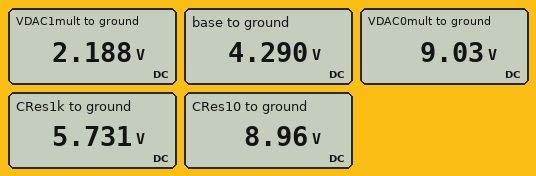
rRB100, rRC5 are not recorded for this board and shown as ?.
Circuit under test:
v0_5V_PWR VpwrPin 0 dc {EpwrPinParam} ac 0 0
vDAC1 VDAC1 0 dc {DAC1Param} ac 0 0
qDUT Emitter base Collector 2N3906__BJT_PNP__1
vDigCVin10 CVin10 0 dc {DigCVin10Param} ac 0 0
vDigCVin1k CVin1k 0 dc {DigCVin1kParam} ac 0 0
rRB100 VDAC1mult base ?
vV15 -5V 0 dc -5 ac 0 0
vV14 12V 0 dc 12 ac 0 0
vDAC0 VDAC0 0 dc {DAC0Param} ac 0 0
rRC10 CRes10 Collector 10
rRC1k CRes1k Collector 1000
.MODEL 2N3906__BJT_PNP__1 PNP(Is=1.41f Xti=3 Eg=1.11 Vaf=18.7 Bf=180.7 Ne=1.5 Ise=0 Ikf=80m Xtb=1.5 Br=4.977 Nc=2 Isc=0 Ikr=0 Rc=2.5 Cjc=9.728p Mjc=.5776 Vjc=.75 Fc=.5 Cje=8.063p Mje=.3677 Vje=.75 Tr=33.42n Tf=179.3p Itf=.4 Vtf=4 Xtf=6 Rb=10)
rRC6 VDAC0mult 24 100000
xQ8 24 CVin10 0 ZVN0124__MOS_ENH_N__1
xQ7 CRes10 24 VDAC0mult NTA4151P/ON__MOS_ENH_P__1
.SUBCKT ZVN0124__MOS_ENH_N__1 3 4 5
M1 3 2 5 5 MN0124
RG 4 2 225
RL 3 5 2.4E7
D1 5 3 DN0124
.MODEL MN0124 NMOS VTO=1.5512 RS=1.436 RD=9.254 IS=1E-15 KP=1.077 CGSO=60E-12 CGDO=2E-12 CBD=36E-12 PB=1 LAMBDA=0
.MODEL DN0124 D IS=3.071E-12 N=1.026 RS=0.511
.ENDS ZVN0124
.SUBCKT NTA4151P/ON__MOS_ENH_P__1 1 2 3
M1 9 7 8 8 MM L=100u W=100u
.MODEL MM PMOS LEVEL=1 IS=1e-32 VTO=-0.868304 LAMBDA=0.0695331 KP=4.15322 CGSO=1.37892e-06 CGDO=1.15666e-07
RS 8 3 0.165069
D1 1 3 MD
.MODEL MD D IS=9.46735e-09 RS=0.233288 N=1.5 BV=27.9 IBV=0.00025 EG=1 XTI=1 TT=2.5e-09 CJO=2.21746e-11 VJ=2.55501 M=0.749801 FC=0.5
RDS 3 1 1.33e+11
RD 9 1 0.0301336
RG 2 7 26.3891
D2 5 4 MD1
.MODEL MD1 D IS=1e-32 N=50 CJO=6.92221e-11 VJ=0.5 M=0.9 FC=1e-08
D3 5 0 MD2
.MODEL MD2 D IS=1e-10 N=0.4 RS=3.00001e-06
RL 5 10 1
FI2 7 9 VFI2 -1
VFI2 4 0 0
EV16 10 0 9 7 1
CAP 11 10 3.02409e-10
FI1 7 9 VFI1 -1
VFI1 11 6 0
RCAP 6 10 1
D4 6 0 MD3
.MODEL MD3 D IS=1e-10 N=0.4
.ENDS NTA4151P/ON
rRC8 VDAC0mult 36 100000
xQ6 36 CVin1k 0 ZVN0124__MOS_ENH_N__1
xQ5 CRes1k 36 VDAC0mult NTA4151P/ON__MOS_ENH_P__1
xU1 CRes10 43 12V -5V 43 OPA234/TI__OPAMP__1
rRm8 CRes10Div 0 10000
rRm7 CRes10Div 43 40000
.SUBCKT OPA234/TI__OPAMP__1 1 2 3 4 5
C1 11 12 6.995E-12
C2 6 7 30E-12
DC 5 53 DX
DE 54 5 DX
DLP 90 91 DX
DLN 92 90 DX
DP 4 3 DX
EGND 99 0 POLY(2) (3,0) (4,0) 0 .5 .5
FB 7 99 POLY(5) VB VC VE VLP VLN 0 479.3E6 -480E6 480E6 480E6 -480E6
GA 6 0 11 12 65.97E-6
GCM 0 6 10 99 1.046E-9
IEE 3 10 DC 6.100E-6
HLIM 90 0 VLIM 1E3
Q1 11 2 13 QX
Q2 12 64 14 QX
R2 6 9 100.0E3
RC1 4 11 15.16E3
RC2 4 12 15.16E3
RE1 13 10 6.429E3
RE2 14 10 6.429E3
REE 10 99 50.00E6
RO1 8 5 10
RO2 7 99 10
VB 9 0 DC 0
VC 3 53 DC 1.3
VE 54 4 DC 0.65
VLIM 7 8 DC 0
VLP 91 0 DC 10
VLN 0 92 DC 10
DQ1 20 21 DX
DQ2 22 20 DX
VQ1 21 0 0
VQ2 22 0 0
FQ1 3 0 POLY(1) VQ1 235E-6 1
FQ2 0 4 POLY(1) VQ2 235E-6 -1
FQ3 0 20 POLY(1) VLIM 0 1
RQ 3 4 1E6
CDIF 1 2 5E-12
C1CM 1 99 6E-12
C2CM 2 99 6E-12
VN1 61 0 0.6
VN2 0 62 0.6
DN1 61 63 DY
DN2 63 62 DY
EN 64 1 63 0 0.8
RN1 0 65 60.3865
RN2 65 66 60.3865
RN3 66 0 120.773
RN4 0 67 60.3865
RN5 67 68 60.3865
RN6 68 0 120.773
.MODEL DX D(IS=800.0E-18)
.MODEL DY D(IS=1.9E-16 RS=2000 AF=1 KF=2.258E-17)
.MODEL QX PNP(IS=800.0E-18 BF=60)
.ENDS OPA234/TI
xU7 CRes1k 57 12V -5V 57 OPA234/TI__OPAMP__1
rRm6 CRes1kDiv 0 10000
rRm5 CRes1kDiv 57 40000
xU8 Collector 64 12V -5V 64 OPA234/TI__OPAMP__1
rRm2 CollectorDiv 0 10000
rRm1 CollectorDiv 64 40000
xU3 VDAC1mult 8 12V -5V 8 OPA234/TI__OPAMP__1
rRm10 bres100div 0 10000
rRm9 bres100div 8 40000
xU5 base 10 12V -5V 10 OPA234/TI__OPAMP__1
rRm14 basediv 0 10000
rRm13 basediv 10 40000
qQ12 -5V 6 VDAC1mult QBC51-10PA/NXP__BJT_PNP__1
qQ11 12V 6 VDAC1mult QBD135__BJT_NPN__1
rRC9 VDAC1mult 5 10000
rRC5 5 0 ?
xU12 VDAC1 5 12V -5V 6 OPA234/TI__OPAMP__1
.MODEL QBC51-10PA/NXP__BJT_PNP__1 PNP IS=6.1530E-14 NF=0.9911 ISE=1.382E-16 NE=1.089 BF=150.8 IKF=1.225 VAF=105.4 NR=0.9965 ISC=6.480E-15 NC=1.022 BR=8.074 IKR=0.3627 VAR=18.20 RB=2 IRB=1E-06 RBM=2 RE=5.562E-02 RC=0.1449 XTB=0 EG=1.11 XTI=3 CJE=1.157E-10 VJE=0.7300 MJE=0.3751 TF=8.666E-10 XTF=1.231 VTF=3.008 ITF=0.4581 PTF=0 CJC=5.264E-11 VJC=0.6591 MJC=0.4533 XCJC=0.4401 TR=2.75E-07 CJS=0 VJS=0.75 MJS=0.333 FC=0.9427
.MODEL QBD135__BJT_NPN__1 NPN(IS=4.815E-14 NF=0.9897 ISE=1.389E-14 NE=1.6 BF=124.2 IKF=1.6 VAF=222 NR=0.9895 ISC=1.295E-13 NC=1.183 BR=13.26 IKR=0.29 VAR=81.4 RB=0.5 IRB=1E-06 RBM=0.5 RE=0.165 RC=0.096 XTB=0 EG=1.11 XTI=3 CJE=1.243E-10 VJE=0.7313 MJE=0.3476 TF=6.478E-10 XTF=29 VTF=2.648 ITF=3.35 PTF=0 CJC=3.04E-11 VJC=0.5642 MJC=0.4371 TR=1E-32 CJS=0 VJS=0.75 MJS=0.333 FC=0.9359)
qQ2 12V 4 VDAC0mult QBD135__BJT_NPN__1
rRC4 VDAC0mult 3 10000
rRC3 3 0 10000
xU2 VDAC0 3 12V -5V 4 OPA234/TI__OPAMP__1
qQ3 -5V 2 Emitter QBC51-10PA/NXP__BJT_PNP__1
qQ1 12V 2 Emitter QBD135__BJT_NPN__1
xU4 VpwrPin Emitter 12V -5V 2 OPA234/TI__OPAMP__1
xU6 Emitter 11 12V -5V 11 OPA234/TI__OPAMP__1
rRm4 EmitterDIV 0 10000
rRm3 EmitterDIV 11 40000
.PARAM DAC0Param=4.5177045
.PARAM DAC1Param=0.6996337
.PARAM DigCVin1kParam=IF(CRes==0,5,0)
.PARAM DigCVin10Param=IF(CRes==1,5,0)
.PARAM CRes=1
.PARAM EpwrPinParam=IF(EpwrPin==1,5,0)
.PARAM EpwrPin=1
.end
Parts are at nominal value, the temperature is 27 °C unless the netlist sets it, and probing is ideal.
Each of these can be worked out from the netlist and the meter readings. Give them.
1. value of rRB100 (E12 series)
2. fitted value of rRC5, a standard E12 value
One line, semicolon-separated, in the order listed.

39 Ω; 4.7 kΩ
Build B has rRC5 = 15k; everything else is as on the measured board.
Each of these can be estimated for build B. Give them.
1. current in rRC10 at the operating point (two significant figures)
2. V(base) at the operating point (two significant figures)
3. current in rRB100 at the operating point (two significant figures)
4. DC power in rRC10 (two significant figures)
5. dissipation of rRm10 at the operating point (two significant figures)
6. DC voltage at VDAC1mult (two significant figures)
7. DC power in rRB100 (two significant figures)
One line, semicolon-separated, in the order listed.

330 mA; 4.0 V; 74 mA; 1.1 W; 5.4 µW; 1.2 V; 210 mW
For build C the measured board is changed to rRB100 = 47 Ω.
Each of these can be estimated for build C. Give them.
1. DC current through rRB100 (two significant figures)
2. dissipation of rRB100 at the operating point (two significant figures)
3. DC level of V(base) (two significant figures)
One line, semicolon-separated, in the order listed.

47 mA; 100 mW; 4.4 V
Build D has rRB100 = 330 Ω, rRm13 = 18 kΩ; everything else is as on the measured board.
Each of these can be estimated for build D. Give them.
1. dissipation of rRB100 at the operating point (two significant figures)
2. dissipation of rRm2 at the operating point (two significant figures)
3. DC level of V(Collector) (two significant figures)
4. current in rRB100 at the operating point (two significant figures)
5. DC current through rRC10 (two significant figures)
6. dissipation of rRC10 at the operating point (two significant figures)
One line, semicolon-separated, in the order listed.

23 mW; 140 µW; 5.9 V; 8.4 mA; 300 mA; 920 mW
